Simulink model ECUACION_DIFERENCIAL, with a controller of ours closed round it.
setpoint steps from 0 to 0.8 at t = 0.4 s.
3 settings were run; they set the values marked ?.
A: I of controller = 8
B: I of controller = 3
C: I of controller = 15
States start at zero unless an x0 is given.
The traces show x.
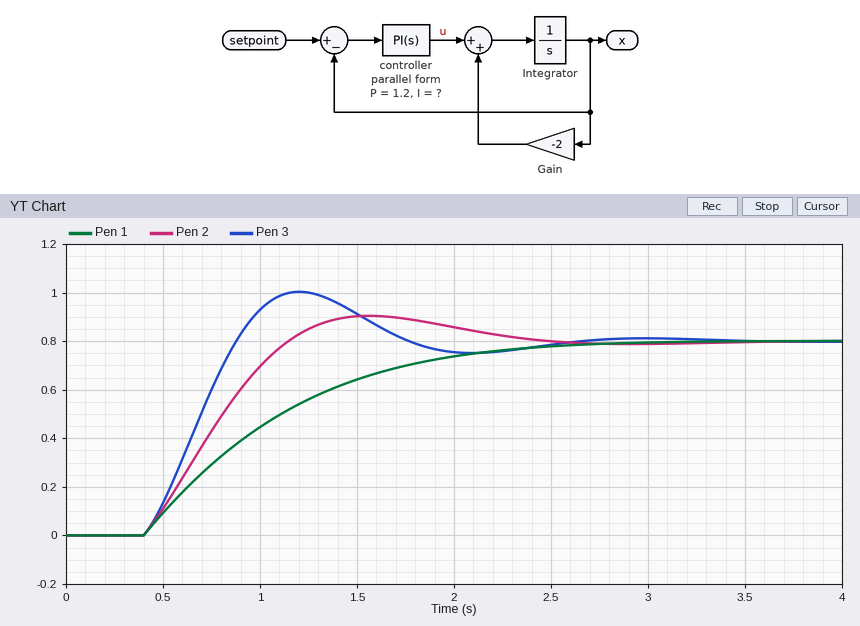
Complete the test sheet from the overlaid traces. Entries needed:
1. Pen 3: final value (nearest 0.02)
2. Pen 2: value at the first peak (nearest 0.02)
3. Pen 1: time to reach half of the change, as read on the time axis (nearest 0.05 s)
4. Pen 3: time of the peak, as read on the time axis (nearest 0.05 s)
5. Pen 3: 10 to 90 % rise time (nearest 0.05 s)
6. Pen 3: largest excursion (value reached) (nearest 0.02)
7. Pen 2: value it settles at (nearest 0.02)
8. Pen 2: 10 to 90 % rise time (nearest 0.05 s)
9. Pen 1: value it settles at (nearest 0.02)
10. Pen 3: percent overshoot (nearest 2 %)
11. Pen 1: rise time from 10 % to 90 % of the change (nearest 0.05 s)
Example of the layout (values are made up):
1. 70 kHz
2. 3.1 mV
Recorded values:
1. 0.80
2. 0.90
3. 0.90 s
4. 1.20 s
5. 0.35 s
6. 1.00
7. 0.80
8. 0.55 s
9. 0.80
10. 26 %
11. 1.40 s
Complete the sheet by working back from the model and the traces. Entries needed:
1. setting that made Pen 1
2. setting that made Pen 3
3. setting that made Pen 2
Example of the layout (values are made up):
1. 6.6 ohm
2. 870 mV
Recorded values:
1. B
2. C
3. A
